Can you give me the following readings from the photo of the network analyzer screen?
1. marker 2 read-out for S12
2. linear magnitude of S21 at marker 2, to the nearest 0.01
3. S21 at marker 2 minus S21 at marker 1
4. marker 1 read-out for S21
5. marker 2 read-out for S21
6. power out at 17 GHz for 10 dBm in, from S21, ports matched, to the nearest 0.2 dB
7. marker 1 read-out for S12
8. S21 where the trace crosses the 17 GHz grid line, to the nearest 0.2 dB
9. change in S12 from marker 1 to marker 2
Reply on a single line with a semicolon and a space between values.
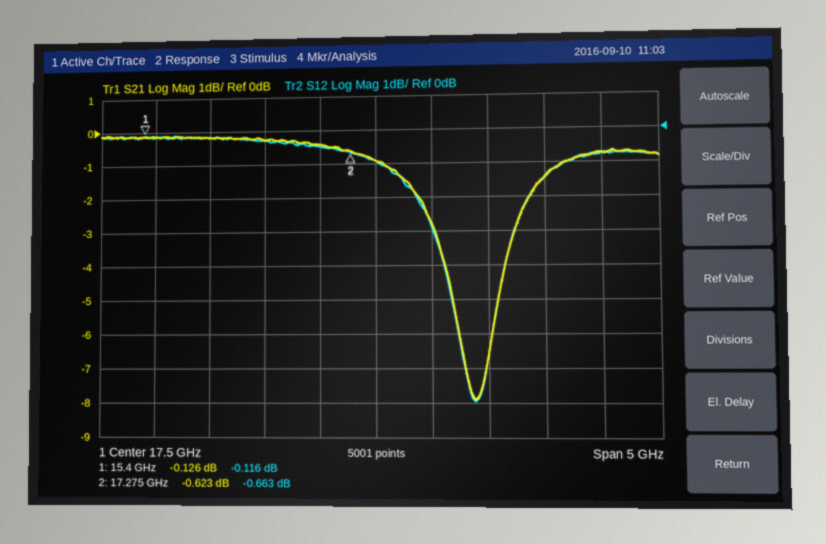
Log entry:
-0.663 dB; 0.93; -0.497 dB; -0.126 dB; -0.623 dB; 9.6 dBm; -0.116 dB; -0.4 dB; -0.547 dB
